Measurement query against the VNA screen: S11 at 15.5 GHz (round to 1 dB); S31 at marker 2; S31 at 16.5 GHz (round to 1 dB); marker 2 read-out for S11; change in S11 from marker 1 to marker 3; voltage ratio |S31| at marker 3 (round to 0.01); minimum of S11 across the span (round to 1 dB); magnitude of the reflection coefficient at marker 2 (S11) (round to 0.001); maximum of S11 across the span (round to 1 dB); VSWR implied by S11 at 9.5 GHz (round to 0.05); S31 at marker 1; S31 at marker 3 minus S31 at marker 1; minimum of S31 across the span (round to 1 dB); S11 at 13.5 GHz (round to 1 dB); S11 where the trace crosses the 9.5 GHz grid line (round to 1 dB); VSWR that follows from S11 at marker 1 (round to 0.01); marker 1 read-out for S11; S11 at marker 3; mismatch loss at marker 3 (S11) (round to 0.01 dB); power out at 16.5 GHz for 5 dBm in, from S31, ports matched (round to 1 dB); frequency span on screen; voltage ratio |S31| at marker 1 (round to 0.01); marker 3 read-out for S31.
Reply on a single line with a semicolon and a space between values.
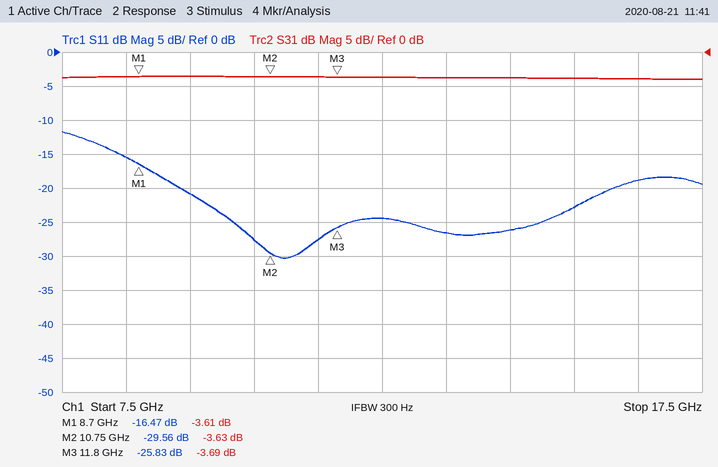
-23 dB; -3.63 dB; -4 dB; -29.56 dB; -9.36 dB; 0.65; -30 dB; 0.033; -12 dB; 1.20; -3.61 dB; -0.08 dB; -4 dB; -27 dB; -21 dB; 1.35; -16.47 dB; -25.83 dB; 0.01 dB; 1 dBm; 10 GHz; 0.66; -3.69 dB
